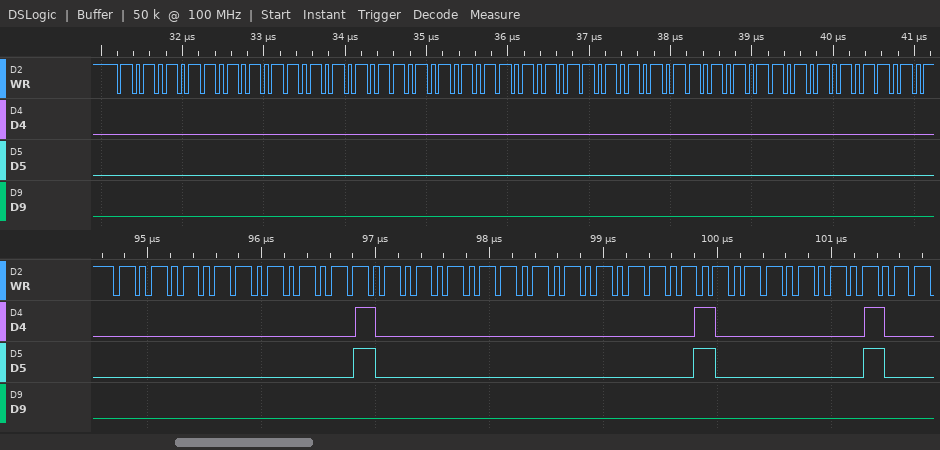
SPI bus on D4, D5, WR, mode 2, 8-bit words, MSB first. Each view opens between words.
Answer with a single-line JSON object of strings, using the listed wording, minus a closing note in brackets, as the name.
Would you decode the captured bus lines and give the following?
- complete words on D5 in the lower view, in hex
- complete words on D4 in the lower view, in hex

{"complete words on D5 in the lower view, in hex": "00, 01, 00, 00, 18, 02", "complete words on D4 in the lower view, in hex": "00, 01, 00, 00, 18, 02"}
